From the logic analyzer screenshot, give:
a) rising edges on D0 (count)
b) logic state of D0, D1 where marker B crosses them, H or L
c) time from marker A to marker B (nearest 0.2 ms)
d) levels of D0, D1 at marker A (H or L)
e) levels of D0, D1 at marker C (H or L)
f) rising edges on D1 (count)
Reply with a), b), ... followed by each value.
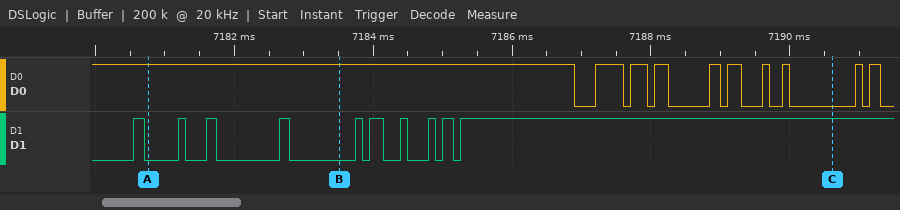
a) 9
b) D0=H, D1=L
c) 2.8 ms
d) D0=H, D1=L
e) D0=L, D1=H
f) 10
